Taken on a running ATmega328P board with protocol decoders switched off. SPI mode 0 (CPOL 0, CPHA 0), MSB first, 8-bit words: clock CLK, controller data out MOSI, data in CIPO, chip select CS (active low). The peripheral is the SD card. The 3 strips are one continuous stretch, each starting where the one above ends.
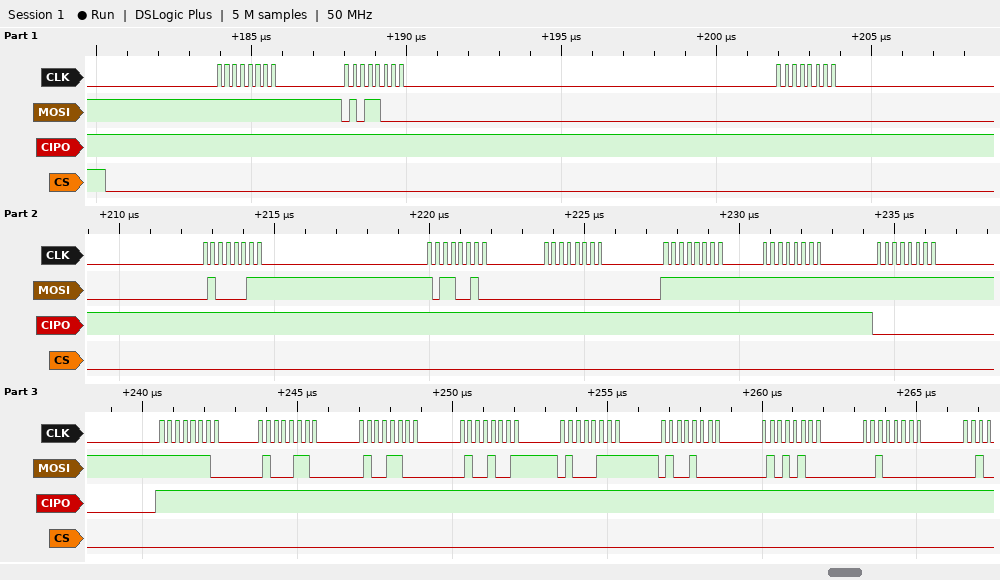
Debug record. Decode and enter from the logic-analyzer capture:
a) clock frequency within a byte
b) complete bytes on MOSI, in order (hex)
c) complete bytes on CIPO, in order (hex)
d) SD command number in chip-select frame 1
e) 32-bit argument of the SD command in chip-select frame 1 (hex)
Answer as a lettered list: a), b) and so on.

a) 4 MHz
b) FF 58 00 43 B2 00 FF FF FF FE 46 4C 49 47 48 54 20
c) FF FF FF FF FF FF FF FF 00 FF FF FF FF FF FF FF FF
d) CMD24
e) 0x0043B200
